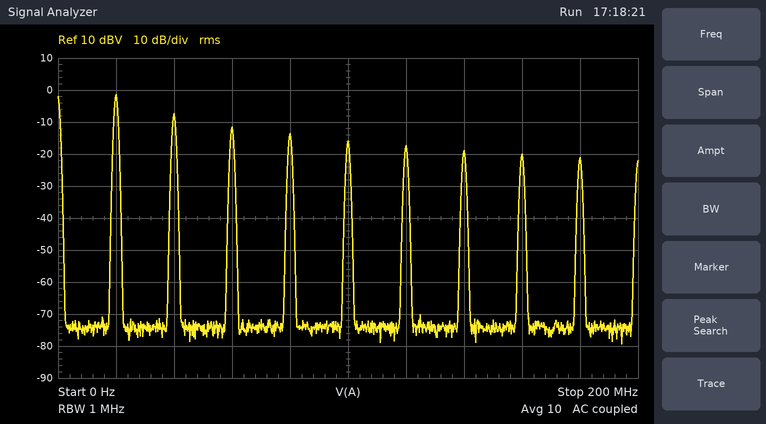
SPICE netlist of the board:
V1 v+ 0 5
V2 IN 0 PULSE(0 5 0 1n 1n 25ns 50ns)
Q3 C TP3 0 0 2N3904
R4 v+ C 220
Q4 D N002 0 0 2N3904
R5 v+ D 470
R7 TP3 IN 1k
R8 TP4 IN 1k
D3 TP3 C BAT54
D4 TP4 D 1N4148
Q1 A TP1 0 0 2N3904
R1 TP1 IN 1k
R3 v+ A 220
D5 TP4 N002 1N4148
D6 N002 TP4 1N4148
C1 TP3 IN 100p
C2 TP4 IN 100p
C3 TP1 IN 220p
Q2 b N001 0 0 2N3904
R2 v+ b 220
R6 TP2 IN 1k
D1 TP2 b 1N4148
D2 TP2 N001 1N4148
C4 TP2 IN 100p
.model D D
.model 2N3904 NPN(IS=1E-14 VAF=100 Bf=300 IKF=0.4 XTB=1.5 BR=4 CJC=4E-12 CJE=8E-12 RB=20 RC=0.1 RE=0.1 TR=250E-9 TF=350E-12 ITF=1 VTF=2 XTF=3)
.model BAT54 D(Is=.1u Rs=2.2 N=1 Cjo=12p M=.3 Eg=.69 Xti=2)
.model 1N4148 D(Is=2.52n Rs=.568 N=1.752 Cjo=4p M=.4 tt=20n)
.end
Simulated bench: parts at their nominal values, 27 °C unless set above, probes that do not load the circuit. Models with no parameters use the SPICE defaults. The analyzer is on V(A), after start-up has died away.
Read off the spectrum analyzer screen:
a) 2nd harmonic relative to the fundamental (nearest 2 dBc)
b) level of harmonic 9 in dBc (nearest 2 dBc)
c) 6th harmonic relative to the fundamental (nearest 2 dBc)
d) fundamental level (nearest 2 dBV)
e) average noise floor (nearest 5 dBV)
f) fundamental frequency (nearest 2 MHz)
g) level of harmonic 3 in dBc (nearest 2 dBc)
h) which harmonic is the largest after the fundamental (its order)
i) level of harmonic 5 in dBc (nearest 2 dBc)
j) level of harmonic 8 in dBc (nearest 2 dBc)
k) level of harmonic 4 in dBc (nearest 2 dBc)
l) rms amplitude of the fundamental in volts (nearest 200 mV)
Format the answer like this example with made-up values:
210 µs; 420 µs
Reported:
-6 dBc; -20 dBc; -16 dBc; -2 dBV; -75 dBV; 20 MHz; -10 dBc; 2; -14 dBc; -18 dBc; -12 dBc; 800 mV
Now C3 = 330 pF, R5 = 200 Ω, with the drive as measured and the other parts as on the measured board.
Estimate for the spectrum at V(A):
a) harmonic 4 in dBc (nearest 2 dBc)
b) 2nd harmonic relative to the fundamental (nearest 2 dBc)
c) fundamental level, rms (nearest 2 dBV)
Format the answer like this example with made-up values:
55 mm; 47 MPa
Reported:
-16 dBc; -10 dBc; 0 dBV
